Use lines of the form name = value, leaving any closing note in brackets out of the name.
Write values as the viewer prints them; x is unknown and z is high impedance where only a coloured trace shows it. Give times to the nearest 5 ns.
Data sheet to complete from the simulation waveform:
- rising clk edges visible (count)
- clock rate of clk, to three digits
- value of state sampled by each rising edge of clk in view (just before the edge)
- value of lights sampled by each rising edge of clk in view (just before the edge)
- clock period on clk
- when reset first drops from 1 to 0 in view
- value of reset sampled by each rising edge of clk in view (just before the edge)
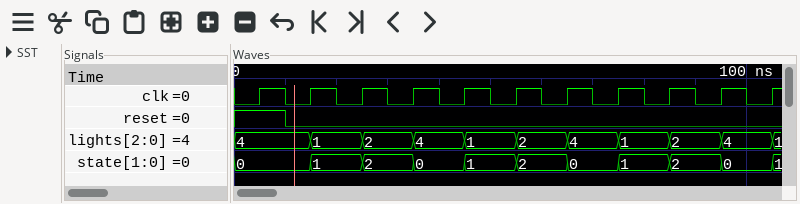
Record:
rising clk edges visible = 11
clock rate of clk, to three digits = 100 MHz
value of state sampled by each rising edge of clk in view = 0, 0, 1, 2, 0, 1, 2, 0, 1, 2, 0
value of lights sampled by each rising edge of clk in view = 4, 4, 1, 2, 4, 1, 2, 4, 1, 2, 4
clock period on clk = 10 ns
when reset first drops from 1 to 0 in view = 10 ns
value of reset sampled by each rising edge of clk in view = 1 0 0 0 0 0 0 0 0 0 0
